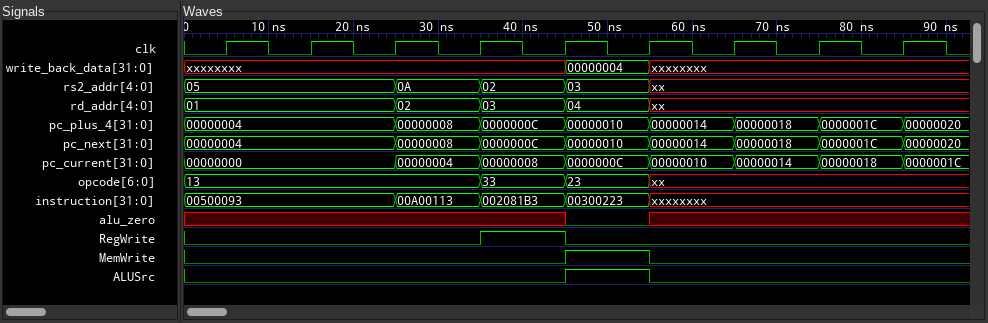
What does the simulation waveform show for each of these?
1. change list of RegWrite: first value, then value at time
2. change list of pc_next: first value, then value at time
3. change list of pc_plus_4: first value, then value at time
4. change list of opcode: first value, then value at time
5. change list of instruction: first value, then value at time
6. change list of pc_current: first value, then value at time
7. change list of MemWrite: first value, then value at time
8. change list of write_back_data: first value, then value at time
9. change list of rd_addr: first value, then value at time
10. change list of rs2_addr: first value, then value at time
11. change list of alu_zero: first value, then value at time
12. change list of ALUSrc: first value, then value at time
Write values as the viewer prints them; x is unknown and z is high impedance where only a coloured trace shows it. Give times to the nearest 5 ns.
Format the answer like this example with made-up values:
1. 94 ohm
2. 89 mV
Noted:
1. 0, 1 at 35 ns, 0 at 45 ns
2. 00000004, 00000008 at 25 ns, 0000000C at 35 ns, 00000010 at 45 ns, 00000014 at 55 ns, 00000018 at 65 ns, 0000001C at 75 ns, 00000020 at 85 ns
3. 00000004, 00000008 at 25 ns, 0000000C at 35 ns, 00000010 at 45 ns, 00000014 at 55 ns, 00000018 at 65 ns, 0000001C at 75 ns, 00000020 at 85 ns
4. 13, 33 at 35 ns, 23 at 45 ns, xx at 55 ns
5. 00500093, 00A00113 at 25 ns, 002081B3 at 35 ns, 00300223 at 45 ns, xxxxxxxx at 55 ns
6. 00000000, 00000004 at 25 ns, 00000008 at 35 ns, 0000000C at 45 ns, 00000010 at 55 ns, 00000014 at 65 ns, 00000018 at 75 ns, 0000001C at 85 ns
7. 0, 1 at 45 ns, 0 at 55 ns
8. xxxxxxxx, 00000004 at 45 ns, xxxxxxxx at 55 ns
9. 01, 02 at 25 ns, 03 at 35 ns, 04 at 45 ns, xx at 55 ns
10. 05, 0A at 25 ns, 02 at 35 ns, 03 at 45 ns, xx at 55 ns
11. x, 0 at 45 ns, x at 55 ns
12. 0, 1 at 45 ns, 0 at 55 ns
